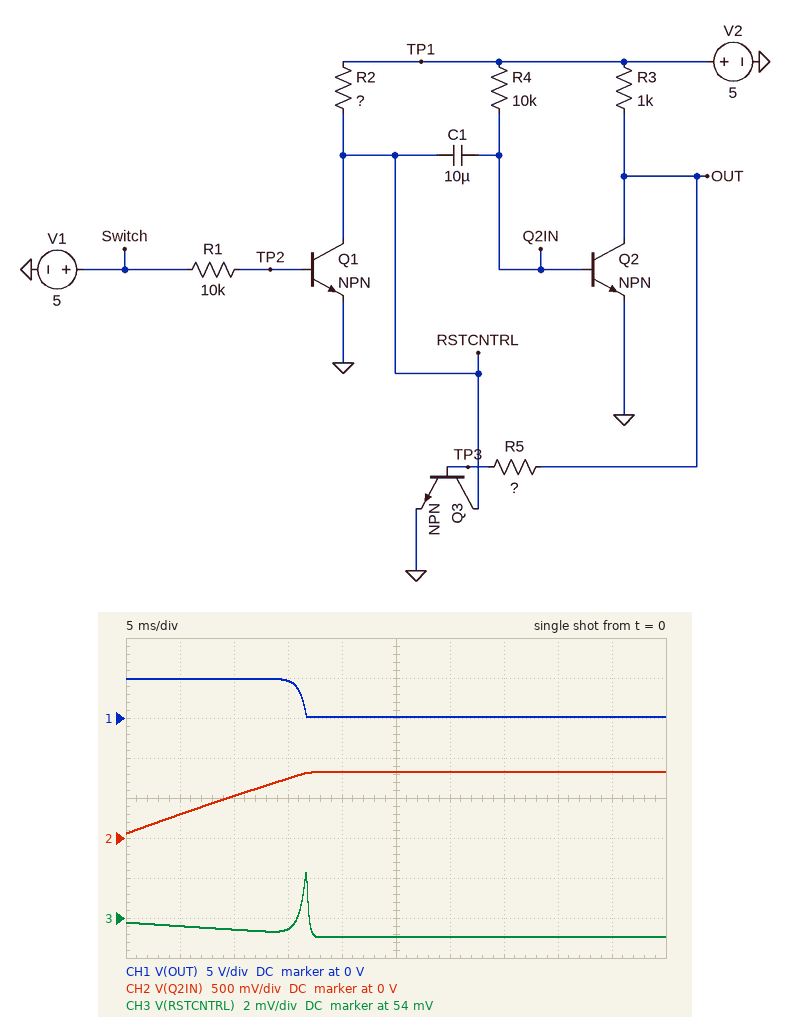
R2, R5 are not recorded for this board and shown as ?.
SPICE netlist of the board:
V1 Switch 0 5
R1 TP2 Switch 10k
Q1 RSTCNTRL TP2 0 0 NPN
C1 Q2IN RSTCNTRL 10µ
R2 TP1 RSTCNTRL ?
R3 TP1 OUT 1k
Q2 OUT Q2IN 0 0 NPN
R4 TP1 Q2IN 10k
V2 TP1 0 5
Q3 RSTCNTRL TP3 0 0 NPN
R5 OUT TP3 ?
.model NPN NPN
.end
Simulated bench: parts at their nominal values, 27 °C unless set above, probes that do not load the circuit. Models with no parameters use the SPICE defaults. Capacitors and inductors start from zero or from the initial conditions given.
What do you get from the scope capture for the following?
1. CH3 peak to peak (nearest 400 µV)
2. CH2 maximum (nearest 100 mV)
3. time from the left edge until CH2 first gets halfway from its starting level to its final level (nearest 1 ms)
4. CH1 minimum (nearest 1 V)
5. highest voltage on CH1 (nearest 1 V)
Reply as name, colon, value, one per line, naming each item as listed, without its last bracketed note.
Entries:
CH3 peak to peak: 3.2 mV
CH2 maximum: 800 mV
time from the left edge until CH2 first gets halfway from its starting level to its final level: 8 ms
CH1 minimum: 0 V
highest voltage on CH1: 5 V
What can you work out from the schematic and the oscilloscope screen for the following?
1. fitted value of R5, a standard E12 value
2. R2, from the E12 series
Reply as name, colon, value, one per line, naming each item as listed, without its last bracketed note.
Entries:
fitted value of R5, a standard E12 value: 56 kΩ
R2, from the E12 series: 2.2 kΩ
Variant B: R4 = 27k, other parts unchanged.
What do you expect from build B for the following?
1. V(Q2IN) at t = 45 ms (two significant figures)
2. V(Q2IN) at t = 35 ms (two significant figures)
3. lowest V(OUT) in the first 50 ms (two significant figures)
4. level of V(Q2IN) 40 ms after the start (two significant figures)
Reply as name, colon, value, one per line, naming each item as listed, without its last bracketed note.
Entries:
V(Q2IN) at t = 45 ms: 810 mV
V(Q2IN) at t = 35 ms: 650 mV
lowest V(OUT) in the first 50 ms: 100 mV
level of V(Q2IN) 40 ms after the start: 730 mV
